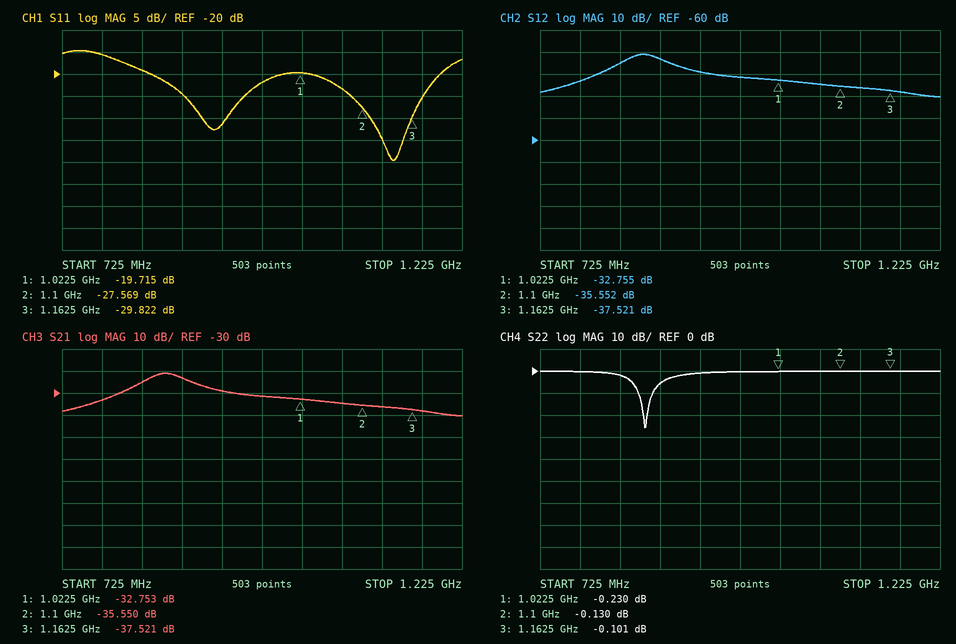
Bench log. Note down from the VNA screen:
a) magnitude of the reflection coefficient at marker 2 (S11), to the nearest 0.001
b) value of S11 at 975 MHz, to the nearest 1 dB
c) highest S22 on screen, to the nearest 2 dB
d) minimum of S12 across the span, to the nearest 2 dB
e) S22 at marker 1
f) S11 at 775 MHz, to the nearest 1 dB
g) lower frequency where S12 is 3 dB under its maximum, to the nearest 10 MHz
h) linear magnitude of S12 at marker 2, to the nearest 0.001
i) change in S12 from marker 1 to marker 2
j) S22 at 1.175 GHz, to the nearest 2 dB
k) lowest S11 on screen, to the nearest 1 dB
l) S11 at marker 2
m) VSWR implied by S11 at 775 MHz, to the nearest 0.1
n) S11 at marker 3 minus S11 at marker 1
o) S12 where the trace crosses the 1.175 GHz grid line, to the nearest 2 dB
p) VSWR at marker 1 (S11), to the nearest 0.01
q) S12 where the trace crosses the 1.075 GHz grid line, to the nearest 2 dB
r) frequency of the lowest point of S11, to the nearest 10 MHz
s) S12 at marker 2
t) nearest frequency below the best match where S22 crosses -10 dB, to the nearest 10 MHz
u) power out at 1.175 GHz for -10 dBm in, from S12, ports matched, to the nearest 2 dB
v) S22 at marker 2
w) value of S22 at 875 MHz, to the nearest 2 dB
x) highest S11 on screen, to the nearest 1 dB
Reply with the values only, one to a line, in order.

0.042
-22 dB
0 dB
-40 dB
-0.230 dB
-16 dB
830 MHz
0.017
-2.797 dB
0 dB
-40 dB
-27.569 dB
1.4
-10.107 dB
-38 dB
1.23
-34 dB
1.14 GHz
-35.552 dB
850 MHz
-48 dBm
-0.130 dB
-6 dB
-15 dB
